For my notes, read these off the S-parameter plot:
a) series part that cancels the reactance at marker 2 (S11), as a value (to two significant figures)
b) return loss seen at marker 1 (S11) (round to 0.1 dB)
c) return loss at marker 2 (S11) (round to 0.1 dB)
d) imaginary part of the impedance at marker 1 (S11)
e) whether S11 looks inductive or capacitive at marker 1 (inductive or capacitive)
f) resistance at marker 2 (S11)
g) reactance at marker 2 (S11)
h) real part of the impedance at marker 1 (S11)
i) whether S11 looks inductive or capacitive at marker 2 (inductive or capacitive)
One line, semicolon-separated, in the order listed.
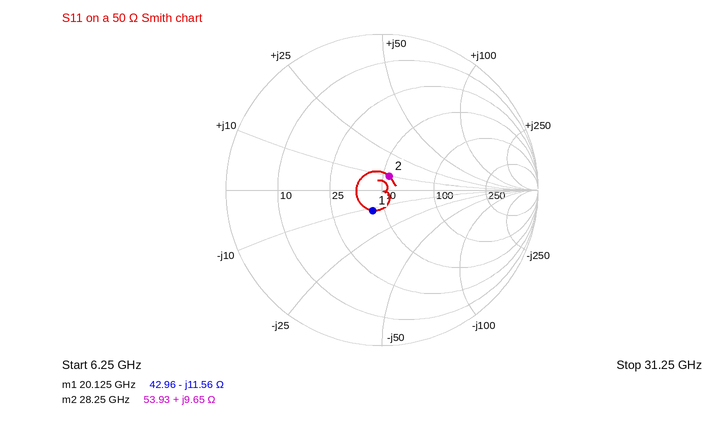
580 fF; 16.8 dB; 20.0 dB; -11.56 Ω; capacitive; 53.93 Ω; +9.65 Ω; 42.96 Ω; inductive
